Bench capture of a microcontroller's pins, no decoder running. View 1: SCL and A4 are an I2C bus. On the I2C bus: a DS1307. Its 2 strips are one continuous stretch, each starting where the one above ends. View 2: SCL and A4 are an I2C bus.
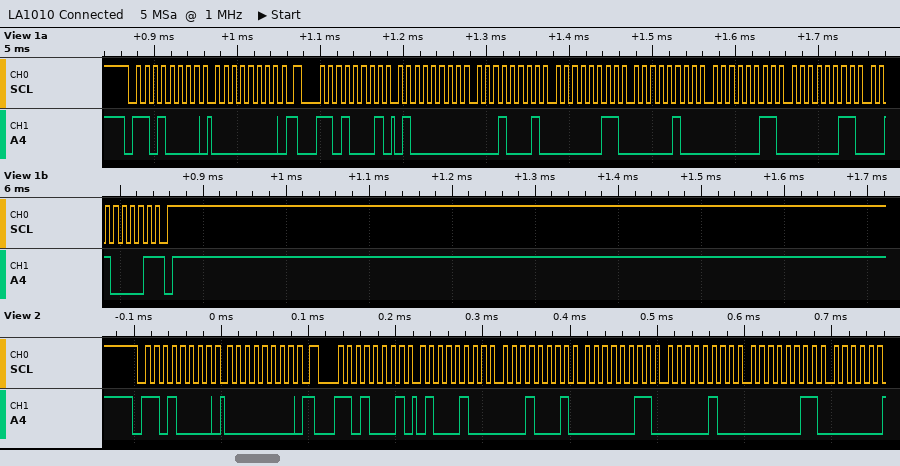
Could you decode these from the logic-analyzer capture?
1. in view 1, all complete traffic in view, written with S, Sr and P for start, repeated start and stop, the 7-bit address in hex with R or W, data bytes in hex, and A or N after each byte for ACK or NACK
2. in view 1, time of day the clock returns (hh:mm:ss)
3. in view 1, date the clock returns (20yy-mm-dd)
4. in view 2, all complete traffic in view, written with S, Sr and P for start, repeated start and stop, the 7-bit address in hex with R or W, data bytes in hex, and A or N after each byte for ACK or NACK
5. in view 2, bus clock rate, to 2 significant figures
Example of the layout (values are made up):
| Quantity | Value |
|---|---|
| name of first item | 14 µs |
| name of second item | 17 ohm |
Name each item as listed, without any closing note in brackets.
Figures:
| Quantity | Value |
|---|---|
| in view 1, all complete traffic in view, written with S, Sr and P for start, repeated start and stop, the 7-bit address in hex with R or W, data bytes in hex, and A or N after each byte for ACK or NACK | S 68W A 00 A Sr 68R A 40 A 11 A 03 A 04 A 03 A 03 A 21 N P |
| in view 1, time of day the clock returns | 03:11:40 |
| in view 1, date the clock returns | 2021-03-03 |
| in view 2, all complete traffic in view, written with S, Sr and P for start, repeated start and stop, the 7-bit address in hex with R or W, data bytes in hex, and A or N after each byte for ACK or NACK | S 68W A 00 A Sr 68R A 44 A 11 A 03 A 04 A 03 A |
| in view 2, bus clock rate, to 2 significant figures | 100 kHz |
